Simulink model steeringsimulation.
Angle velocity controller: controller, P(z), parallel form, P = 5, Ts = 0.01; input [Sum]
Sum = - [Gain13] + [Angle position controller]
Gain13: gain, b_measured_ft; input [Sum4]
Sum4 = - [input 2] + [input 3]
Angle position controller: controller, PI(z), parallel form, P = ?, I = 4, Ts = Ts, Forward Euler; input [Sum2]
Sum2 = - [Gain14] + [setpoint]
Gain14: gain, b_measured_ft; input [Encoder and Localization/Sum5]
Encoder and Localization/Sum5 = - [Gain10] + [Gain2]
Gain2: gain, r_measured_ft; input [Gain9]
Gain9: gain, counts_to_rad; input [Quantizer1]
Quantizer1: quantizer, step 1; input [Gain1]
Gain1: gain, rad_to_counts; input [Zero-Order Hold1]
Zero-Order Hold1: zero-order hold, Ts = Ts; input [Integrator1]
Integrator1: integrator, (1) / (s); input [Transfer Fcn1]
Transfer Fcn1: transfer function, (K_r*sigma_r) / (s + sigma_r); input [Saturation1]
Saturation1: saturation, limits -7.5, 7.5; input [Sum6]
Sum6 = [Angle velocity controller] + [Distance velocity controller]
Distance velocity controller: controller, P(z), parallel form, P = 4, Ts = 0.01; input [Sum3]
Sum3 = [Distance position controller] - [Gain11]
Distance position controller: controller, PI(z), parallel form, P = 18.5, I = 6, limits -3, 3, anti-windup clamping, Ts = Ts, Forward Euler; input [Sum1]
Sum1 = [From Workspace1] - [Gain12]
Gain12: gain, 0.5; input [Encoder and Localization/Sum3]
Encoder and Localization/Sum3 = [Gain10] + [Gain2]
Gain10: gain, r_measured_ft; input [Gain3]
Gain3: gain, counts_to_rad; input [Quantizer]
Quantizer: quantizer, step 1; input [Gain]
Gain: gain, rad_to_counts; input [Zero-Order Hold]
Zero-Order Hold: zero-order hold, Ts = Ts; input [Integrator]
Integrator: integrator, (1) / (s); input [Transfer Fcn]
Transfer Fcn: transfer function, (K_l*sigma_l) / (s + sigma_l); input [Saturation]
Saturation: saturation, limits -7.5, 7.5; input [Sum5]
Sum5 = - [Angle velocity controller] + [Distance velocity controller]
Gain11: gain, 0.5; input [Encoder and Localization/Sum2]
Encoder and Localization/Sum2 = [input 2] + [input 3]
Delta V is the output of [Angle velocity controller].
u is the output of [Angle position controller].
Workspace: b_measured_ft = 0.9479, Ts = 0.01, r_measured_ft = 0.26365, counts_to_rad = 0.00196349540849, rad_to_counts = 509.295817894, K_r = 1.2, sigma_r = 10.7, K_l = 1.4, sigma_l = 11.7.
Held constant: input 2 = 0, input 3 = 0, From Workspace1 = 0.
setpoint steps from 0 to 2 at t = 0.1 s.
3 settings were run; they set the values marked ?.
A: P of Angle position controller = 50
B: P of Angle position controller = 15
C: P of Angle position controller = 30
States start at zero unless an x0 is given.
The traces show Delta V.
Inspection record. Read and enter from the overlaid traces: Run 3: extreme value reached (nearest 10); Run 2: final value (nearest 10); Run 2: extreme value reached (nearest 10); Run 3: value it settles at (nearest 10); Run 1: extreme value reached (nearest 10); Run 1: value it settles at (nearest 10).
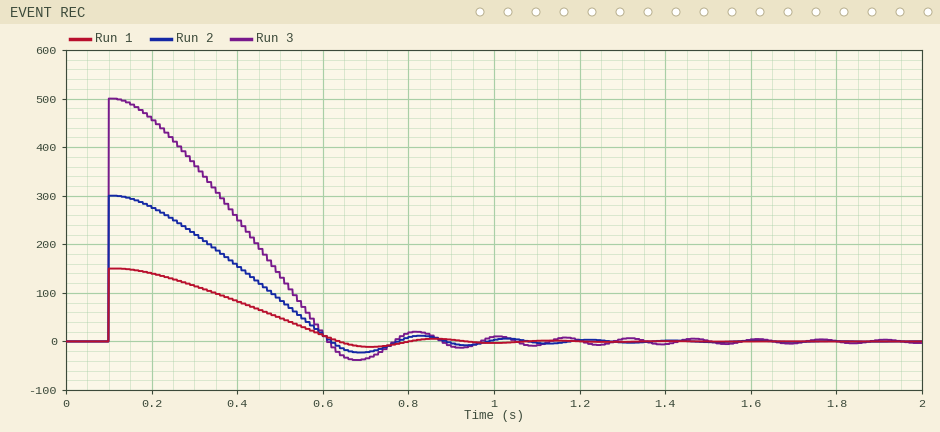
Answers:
500
0
300
0
150
0
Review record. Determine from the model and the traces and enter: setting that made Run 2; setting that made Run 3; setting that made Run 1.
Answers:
C
A
B
